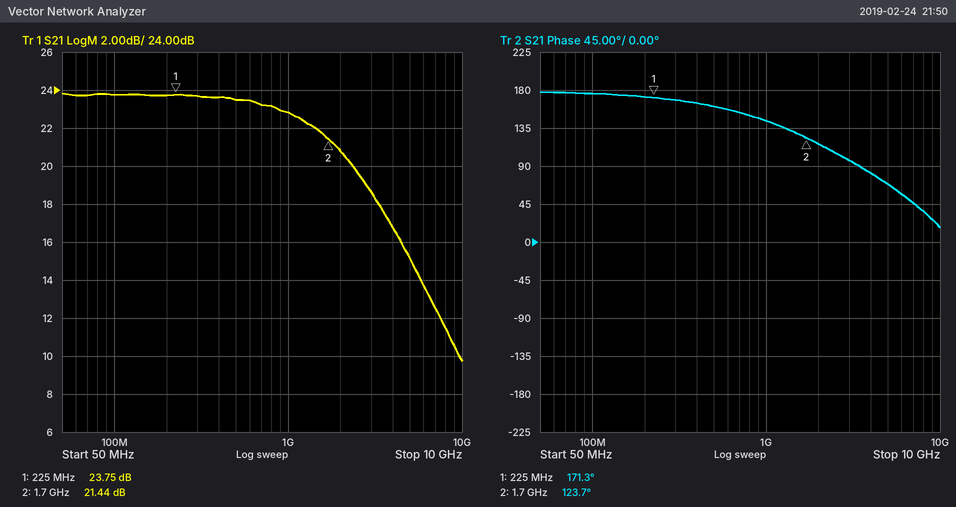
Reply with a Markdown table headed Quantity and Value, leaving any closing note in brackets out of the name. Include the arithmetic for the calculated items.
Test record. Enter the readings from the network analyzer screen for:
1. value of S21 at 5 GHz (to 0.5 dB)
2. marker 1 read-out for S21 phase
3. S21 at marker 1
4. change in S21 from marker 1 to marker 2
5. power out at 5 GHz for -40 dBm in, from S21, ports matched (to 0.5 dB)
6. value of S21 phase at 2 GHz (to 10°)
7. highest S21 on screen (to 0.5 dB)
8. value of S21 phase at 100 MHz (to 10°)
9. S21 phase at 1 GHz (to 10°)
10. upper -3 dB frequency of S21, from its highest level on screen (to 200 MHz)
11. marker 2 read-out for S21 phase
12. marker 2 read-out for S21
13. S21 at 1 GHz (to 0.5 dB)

| Quantity | Value |
|---|---|
| value of S21 at 5 GHz | 15.0 dB |
| marker 1 read-out for S21 phase | 171.3° |
| S21 at marker 1 | 23.75 dB |
| change in S21 from marker 1 to marker 2 | 21.44 − (23.75) = -2.31 dB |
| power out at 5 GHz for -40 dBm in, from S21, ports matched | -40 dBm + (15.0 dB) = -25.0 dBm |
| value of S21 phase at 2 GHz | 120° |
| highest S21 on screen | 24.0 dB |
| value of S21 phase at 100 MHz | 180° |
| S21 phase at 1 GHz | 140° |
| upper -3 dB frequency of S21, from its highest level on screen | 2.0 GHz |
| marker 2 read-out for S21 phase | 123.7° |
| marker 2 read-out for S21 | 21.44 dB |
| S21 at 1 GHz | 23.0 dB |
